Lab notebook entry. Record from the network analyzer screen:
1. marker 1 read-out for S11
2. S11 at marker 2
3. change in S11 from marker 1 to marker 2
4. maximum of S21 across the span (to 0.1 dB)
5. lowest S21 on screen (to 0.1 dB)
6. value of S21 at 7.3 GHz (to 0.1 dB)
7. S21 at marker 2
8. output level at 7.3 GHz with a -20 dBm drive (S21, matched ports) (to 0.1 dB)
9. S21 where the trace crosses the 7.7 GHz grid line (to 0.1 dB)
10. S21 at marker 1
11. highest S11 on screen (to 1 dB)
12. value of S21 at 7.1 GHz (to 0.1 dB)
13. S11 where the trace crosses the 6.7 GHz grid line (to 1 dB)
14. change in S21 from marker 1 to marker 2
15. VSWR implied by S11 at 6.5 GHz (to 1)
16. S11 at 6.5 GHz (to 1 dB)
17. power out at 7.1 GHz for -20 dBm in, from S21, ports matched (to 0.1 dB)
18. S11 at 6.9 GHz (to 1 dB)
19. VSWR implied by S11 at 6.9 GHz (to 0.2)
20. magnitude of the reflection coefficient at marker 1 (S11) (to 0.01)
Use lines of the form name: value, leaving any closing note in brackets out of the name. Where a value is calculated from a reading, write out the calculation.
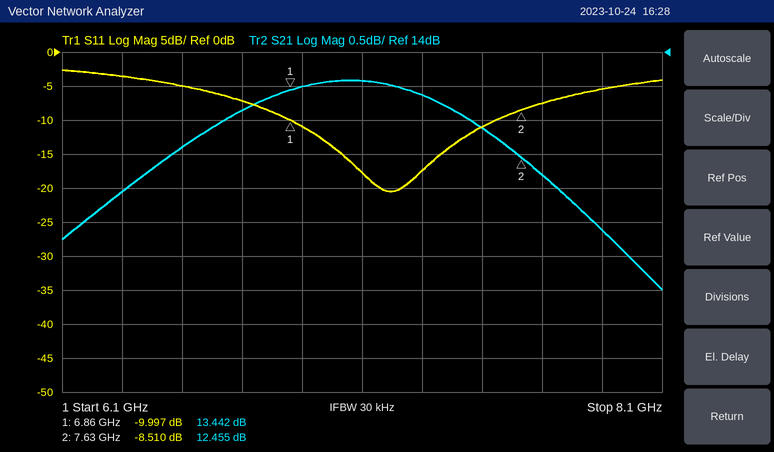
marker 1 read-out for S11: -9.997 dB
S11 at marker 2: -8.510 dB
change in S11 from marker 1 to marker 2: -8.51 − (-9.997) = 1.487 dB
maximum of S21 across the span: 13.6 dB
lowest S21 on screen: 10.5 dB
value of S21 at 7.3 GHz: 13.4 dB
S21 at marker 2: 12.455 dB
output level at 7.3 GHz with a -20 dBm drive (S21, matched ports): -20 dBm + (13.4 dB) = -6.6 dBm
S21 where the trace crosses the 7.7 GHz grid line: 12.2 dB
S21 at marker 1: 13.442 dB
highest S11 on screen: -3 dB
value of S21 at 7.1 GHz: 13.6 dB
S11 where the trace crosses the 6.7 GHz grid line: -7 dB
change in S21 from marker 1 to marker 2: 12.455 − (13.442) = -0.987 dB
VSWR implied by S11 at 6.5 GHz: |Γ| = 10^(-5/20) = 0.5623; VSWR = (1 + 0.5623)/(1 − 0.5623) ≈ 4
S11 at 6.5 GHz: -5 dB
power out at 7.1 GHz for -20 dBm in, from S21, ports matched: -20 dBm + (13.6 dB) = -6.4 dBm
S11 at 6.9 GHz: -11 dB
VSWR implied by S11 at 6.9 GHz: |Γ| = 10^(-11/20) = 0.2818; VSWR = (1 + 0.2818)/(1 − 0.2818) ≈ 1.8
magnitude of the reflection coefficient at marker 1 (S11): 10^(-9.997/20) ≈ 0.32
